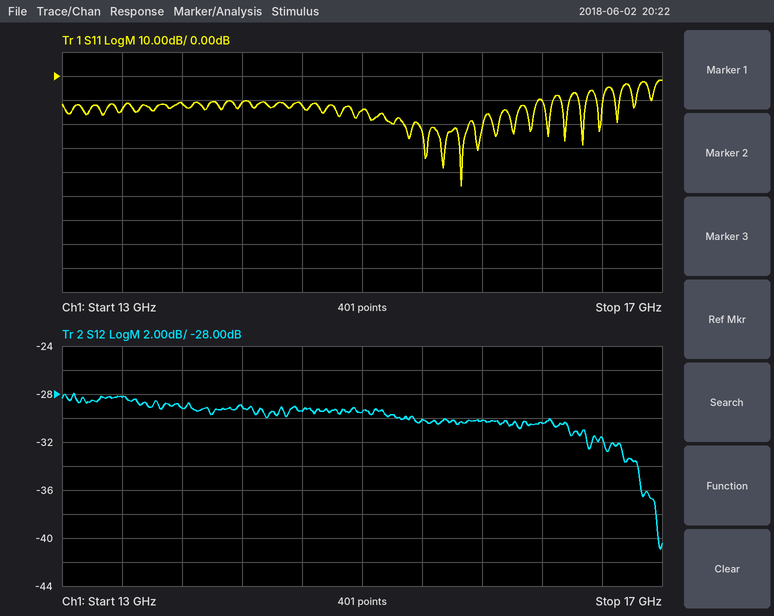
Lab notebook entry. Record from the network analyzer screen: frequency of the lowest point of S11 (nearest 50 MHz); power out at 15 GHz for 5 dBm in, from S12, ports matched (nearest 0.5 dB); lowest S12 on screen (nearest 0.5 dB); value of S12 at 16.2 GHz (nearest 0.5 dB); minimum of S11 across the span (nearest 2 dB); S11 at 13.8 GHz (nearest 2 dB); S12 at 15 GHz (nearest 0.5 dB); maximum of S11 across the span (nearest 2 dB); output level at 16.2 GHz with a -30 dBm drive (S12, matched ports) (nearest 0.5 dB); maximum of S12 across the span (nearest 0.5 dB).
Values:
15.65 GHz
-24.5 dBm
-41.0 dB
-30.5 dB
-46 dB
-12 dB
-29.5 dB
-2 dB
-60.5 dBm
-28.0 dB
